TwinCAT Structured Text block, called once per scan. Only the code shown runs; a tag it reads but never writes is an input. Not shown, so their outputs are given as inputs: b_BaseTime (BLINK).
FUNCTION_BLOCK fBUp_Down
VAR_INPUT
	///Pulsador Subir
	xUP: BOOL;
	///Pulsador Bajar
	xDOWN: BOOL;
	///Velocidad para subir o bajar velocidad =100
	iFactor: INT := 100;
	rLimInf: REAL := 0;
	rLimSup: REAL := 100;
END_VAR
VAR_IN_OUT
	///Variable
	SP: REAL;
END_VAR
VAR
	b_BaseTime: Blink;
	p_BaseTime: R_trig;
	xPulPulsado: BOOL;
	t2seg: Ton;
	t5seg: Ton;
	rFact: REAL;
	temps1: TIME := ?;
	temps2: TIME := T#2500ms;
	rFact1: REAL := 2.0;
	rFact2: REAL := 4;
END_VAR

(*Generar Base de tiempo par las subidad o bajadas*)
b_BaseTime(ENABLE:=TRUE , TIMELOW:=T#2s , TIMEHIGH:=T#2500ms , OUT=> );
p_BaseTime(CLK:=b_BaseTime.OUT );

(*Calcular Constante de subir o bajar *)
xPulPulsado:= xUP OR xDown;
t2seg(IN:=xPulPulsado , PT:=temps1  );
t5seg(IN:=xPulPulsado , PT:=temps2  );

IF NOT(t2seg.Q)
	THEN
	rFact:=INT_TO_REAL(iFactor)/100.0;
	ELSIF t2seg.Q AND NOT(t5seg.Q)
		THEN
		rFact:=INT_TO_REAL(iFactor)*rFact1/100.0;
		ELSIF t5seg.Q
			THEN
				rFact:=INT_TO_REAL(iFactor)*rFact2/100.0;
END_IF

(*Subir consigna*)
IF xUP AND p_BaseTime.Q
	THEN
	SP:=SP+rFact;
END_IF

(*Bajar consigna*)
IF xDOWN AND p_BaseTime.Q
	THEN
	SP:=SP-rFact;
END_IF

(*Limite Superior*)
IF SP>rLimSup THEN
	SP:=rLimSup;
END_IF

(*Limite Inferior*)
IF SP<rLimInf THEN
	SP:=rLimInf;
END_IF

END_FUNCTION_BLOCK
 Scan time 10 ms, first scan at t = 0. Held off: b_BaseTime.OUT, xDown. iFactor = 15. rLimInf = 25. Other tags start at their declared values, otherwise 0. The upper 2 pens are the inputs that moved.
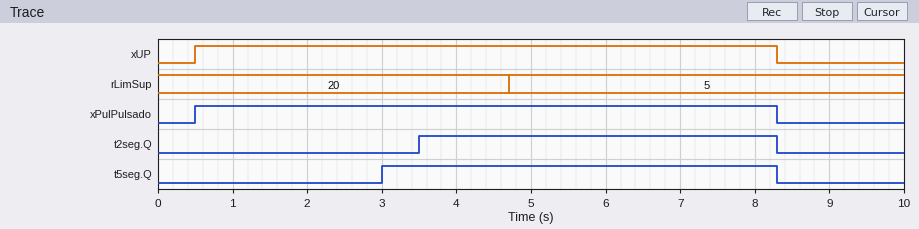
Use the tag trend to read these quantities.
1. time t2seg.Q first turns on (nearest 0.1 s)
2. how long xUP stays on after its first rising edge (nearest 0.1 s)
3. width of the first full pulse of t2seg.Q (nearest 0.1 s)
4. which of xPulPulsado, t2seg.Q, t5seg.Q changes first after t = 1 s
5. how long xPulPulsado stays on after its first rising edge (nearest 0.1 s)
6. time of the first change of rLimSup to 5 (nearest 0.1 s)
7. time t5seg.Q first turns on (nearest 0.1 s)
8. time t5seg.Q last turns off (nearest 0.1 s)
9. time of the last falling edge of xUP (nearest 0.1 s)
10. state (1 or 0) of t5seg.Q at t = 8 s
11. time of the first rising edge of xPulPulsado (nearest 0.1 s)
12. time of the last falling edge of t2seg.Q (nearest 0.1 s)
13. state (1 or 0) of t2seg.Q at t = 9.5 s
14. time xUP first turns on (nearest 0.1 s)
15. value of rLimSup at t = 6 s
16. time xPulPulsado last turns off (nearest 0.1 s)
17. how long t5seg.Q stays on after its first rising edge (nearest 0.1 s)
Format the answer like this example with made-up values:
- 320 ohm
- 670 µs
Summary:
- 3.5 s
- 7.8 s
- 4.8 s
- t5seg.Q
- 7.8 s
- 4.7 s
- 3.0 s
- 8.3 s
- 8.3 s
- 1
- 0.5 s
- 8.3 s
- 0
- 0.5 s
- 5
- 8.3 s
- 5.3 s
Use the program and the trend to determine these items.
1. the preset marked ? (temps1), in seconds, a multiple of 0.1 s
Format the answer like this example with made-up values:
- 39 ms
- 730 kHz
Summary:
- 3.0 s
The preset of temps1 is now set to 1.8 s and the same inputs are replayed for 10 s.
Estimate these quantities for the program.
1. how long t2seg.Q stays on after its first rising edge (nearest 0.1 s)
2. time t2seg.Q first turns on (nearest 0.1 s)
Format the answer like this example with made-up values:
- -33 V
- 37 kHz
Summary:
- 6.0 s
- 2.3 s
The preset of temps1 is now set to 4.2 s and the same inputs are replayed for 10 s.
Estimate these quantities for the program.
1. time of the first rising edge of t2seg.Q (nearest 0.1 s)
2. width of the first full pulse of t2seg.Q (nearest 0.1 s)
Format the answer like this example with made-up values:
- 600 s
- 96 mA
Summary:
- 4.7 s
- 3.6 s
